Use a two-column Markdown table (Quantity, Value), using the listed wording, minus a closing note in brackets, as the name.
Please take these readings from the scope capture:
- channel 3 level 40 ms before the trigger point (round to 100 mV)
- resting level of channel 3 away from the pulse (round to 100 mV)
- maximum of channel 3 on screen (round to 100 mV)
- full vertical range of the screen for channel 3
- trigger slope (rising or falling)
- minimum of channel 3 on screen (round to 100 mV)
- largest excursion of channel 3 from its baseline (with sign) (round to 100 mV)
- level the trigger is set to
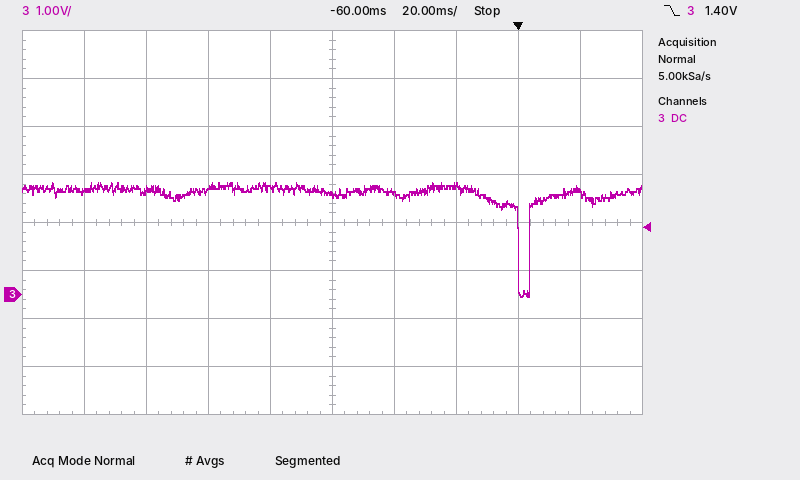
| Quantity | Value |
|---|---|
| channel 3 level 40 ms before the trigger point | 2.1 V |
| resting level of channel 3 away from the pulse | 2.2 V |
| maximum of channel 3 on screen | 2.3 V |
| full vertical range of the screen for channel 3 | 8 V |
| trigger slope | falling |
| minimum of channel 3 on screen | 0.0 V |
| largest excursion of channel 3 from its baseline (with sign) | -2.2 V |
| level the trigger is set to | 1.40 V |
